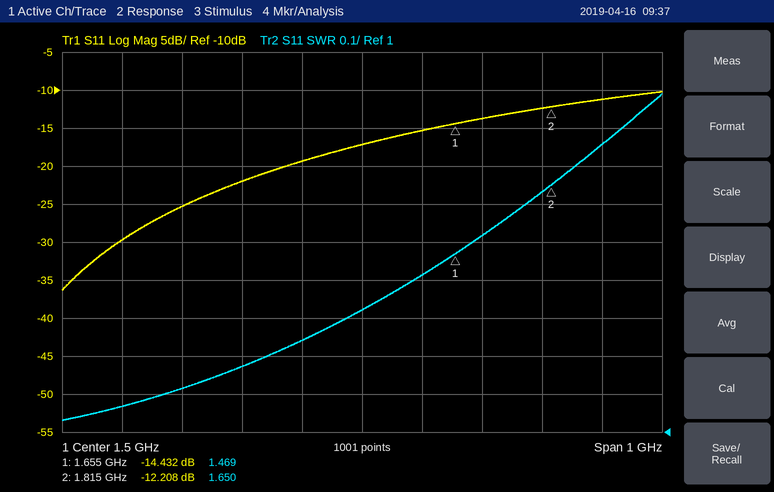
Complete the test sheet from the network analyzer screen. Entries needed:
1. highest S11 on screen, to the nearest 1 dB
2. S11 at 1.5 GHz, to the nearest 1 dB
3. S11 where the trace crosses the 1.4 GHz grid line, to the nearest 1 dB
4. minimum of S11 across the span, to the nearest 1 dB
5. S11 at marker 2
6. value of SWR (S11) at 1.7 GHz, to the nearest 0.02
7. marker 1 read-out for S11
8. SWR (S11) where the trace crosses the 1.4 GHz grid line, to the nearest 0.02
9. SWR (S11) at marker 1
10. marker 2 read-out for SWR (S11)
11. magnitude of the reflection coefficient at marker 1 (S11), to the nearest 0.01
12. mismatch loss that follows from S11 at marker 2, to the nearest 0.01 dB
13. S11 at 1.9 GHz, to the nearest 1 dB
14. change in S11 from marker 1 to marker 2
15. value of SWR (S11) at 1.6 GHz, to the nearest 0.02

-10 dB
-17 dB
-19 dB
-36 dB
-12.208 dB
1.52
-14.432 dB
1.24
1.469
1.650
0.19
0.27 dB
-11 dB
2.224 dB
1.42
